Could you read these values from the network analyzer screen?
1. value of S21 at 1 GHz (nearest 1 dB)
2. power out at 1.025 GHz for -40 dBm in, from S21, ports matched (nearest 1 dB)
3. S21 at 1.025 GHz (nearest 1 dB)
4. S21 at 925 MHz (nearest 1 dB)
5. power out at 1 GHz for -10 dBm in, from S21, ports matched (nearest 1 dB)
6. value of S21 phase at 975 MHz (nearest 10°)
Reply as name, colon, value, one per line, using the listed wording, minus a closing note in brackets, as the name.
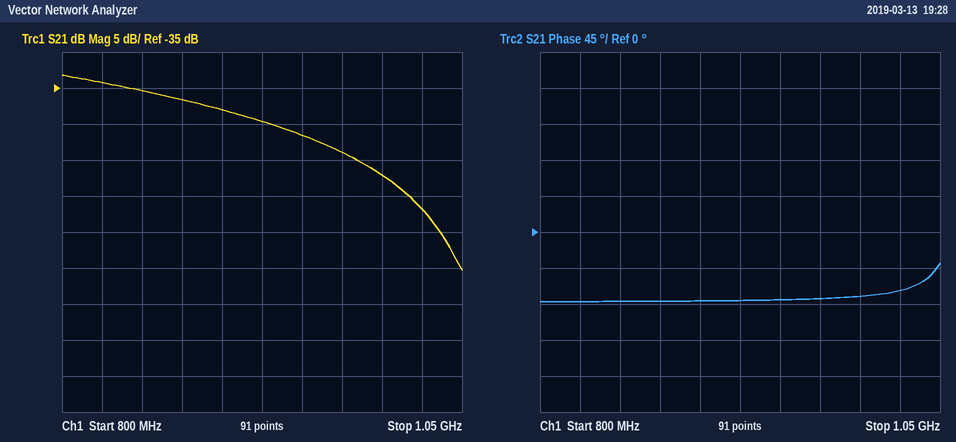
value of S21 at 1 GHz: -47 dB
power out at 1.025 GHz for -40 dBm in, from S21, ports matched: -92 dBm
S21 at 1.025 GHz: -52 dB
S21 at 925 MHz: -40 dB
power out at 1 GHz for -10 dBm in, from S21, ports matched: -57 dBm
value of S21 phase at 975 MHz: -80°
